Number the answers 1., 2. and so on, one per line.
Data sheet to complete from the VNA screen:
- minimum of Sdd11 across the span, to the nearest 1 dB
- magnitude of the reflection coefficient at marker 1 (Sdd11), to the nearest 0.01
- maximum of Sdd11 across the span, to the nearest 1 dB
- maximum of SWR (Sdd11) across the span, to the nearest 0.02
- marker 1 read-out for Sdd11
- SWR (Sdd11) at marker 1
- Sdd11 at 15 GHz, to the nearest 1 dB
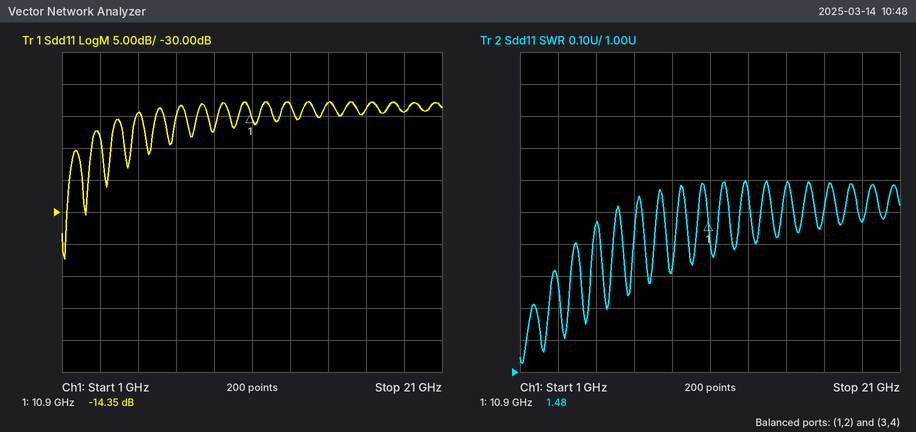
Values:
1. -37 dB
2. 0.19
3. -13 dB
4. 1.60
5. -14.35 dB
6. 1.48
7. -13 dB
